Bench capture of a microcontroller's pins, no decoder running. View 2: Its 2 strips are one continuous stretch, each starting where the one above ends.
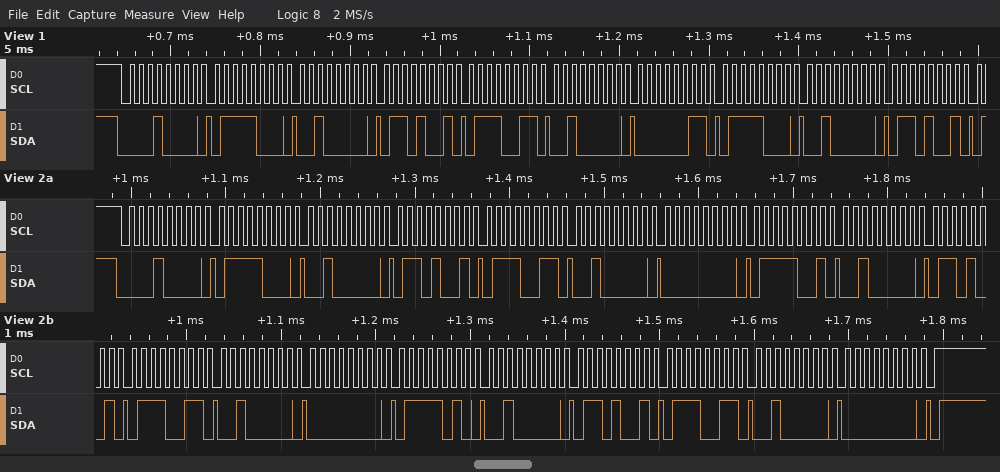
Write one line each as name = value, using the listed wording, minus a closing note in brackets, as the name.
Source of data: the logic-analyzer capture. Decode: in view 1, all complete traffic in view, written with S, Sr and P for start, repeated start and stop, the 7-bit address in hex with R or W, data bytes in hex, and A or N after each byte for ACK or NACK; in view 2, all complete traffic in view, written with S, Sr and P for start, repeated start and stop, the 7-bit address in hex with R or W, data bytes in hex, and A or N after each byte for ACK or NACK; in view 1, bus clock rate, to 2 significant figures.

in view 1, all complete traffic in view, written with S, Sr and P for start, repeated start and stop, the 7-bit address in hex with R or W, data bytes in hex, and A or N after each byte for ACK or NACK = S 08W A 78 A 20 A 69 A 73 A 20 A 03 A 78 A 20 A 69 A
in view 2, all complete traffic in view, written with S, Sr and P for start, repeated start and stop, the 7-bit address in hex with R or W, data bytes in hex, and A or N after each byte for ACK or NACK = S 08W A 78 A 20 A 69 A 73 A 20 A 00 A 79 A 20 A 69 A 73 A 20 A 00 A 7A A 20 A 69 A 73 A 20 A 00 A P
in view 1, bus clock rate, to 2 significant figures = 100 kHz
